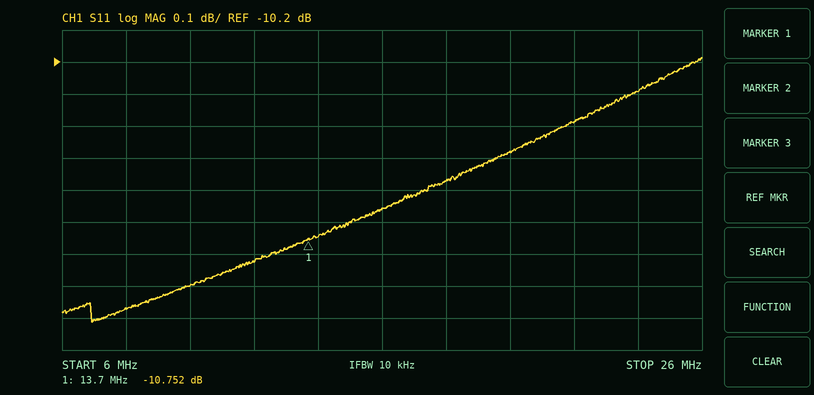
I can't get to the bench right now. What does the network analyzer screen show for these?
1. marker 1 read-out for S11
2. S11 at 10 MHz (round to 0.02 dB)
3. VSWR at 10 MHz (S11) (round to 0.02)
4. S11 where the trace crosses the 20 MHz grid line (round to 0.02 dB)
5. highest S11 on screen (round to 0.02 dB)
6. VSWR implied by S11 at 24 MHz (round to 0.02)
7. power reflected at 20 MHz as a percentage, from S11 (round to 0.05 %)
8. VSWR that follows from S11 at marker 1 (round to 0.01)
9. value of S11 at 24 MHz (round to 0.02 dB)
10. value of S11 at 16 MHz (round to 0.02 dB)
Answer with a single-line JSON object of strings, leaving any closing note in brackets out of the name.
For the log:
{"marker 1 read-out for S11": "-10.752 dB", "S11 at 10 MHz": "-10.90 dB", "VSWR at 10 MHz (S11)": "1.80", "S11 where the trace crosses the 20 MHz grid line": "-10.48 dB", "highest S11 on screen": "-10.18 dB", "VSWR implied by S11 at 24 MHz": "1.88", "power reflected at 20 MHz as a percentage, from S11": "8.95 %", "VSWR that follows from S11 at marker 1": "1.82", "value of S11 at 24 MHz": "-10.30 dB", "value of S11 at 16 MHz": "-10.66 dB"}
